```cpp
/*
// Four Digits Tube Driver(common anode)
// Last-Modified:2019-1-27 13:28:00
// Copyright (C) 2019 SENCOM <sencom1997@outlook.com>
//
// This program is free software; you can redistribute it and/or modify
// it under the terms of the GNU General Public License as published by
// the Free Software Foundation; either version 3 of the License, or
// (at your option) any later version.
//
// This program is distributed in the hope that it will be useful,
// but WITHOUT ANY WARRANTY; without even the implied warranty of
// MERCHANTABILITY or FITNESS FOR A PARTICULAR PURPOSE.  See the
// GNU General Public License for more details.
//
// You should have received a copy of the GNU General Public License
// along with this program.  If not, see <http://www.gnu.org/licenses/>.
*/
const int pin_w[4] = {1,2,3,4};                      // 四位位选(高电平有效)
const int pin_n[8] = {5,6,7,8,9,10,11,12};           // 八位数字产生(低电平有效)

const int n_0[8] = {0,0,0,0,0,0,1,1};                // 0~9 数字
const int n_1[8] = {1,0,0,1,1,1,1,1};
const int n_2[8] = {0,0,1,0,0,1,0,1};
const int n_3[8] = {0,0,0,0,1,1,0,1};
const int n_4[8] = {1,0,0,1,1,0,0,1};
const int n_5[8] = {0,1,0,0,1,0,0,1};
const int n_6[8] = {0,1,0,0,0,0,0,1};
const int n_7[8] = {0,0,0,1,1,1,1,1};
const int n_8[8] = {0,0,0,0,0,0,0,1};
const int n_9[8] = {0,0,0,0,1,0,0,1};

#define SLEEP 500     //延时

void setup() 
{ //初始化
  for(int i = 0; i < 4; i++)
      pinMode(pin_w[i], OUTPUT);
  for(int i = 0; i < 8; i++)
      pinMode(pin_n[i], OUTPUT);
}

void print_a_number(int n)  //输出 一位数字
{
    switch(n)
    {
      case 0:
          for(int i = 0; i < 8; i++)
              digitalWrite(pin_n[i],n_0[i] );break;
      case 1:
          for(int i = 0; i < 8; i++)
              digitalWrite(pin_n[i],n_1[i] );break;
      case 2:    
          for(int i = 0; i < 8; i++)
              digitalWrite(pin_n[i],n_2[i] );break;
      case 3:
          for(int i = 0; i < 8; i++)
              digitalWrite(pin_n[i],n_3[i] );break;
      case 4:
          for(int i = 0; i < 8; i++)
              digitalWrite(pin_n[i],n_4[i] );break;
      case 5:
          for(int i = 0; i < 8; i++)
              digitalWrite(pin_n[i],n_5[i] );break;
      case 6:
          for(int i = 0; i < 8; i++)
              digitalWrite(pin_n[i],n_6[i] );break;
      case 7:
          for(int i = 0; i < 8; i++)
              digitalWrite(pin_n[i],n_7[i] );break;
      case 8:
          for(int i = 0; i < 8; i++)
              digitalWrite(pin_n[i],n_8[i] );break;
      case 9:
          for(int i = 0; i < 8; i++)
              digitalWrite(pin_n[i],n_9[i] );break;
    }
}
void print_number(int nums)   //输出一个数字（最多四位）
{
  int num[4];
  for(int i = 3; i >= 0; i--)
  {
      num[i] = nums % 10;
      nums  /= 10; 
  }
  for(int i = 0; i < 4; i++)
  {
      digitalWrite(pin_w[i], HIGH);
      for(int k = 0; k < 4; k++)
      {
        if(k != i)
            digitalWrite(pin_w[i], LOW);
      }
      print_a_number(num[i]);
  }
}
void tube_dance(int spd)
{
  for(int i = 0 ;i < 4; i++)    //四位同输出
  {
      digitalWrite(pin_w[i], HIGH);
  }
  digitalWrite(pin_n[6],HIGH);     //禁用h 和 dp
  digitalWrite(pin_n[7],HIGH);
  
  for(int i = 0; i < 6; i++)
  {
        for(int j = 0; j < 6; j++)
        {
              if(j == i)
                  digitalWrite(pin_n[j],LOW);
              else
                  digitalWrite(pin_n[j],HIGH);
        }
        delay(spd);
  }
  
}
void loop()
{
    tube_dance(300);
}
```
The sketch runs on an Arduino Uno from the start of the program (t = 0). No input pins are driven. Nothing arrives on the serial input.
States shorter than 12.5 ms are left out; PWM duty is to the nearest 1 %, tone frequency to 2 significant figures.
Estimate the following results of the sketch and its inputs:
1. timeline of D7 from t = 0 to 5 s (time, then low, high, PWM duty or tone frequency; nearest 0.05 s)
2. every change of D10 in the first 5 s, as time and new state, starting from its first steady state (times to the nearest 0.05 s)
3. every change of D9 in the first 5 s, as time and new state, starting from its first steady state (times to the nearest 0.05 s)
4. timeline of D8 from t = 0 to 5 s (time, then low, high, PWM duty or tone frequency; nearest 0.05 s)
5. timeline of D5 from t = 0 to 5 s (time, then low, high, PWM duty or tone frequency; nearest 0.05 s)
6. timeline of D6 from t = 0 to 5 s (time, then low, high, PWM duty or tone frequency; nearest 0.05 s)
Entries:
0 s high; 0.6 s low; 0.9 s high; 2.4 s low; 2.7 s high; 4.2 s low; 4.5 s high
0 s high; 1.5 s low; 1.8 s high; 3.3 s low; 3.6 s high
0 s high; 1.2 s low; 1.5 s high; 3 s low; 3.3 s high; 4.8 s low
0 s high; 0.9 s low; 1.2 s high; 2.7 s low; 3 s high; 4.5 s low; 4.8 s high
0 s low; 0.3 s high; 1.8 s low; 2.1 s high; 3.6 s low; 3.9 s high
0 s high; 0.3 s low; 0.6 s high; 2.1 s low; 2.4 s high; 3.9 s low; 4.2 s high
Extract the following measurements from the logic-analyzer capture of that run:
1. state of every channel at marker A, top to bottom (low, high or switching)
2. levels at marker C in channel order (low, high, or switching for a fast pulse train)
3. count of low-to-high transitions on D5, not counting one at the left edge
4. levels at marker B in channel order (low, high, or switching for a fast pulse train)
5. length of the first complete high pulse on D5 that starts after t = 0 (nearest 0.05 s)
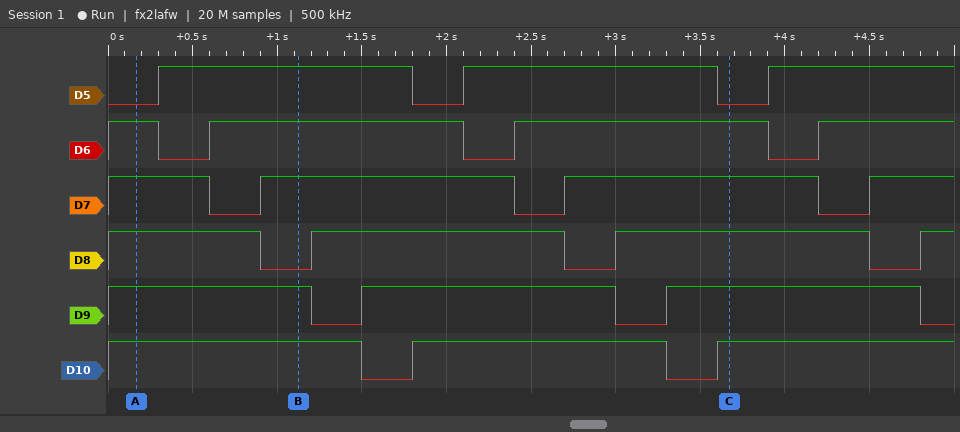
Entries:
D5 low, D6 high, D7 high, D8 high, D9 high, D10 high
D5 low, D6 high, D7 high, D8 high, D9 high, D10 high
3
D5 high, D6 high, D7 high, D8 low, D9 high, D10 high
1.50 s
